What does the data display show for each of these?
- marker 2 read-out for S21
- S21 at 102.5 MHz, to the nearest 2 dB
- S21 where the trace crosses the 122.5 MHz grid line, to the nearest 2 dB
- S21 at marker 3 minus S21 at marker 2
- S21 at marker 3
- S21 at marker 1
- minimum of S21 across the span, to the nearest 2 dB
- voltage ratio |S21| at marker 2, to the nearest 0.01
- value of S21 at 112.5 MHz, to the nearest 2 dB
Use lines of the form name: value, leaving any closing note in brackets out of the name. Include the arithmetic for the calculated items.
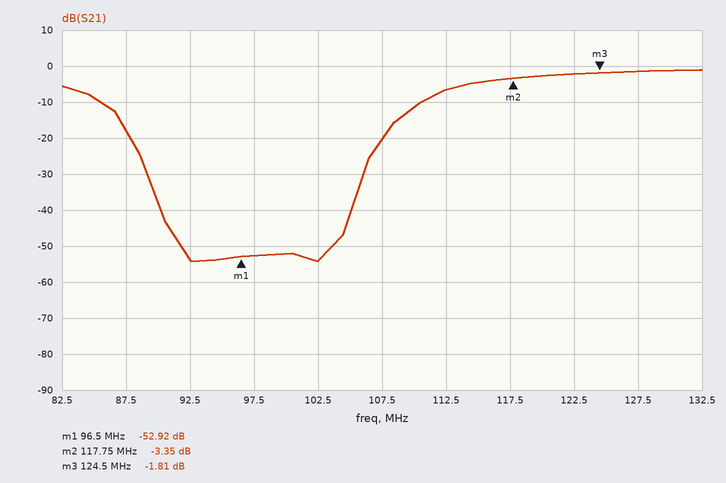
marker 2 read-out for S21: -3.35 dB
S21 at 102.5 MHz, to the nearest 2 dB: -54 dB
S21 where the trace crosses the 122.5 MHz grid line, to the nearest 2 dB: -2 dB
S21 at marker 3 minus S21 at marker 2: -1.81 − (-3.35) = 1.54 dB
S21 at marker 3: -1.81 dB
S21 at marker 1: -52.92 dB
minimum of S21 across the span, to the nearest 2 dB: -54 dB
voltage ratio |S21| at marker 2, to the nearest 0.01: 10^(-3.35/20) ≈ 0.68
value of S21 at 112.5 MHz, to the nearest 2 dB: -6 dB
